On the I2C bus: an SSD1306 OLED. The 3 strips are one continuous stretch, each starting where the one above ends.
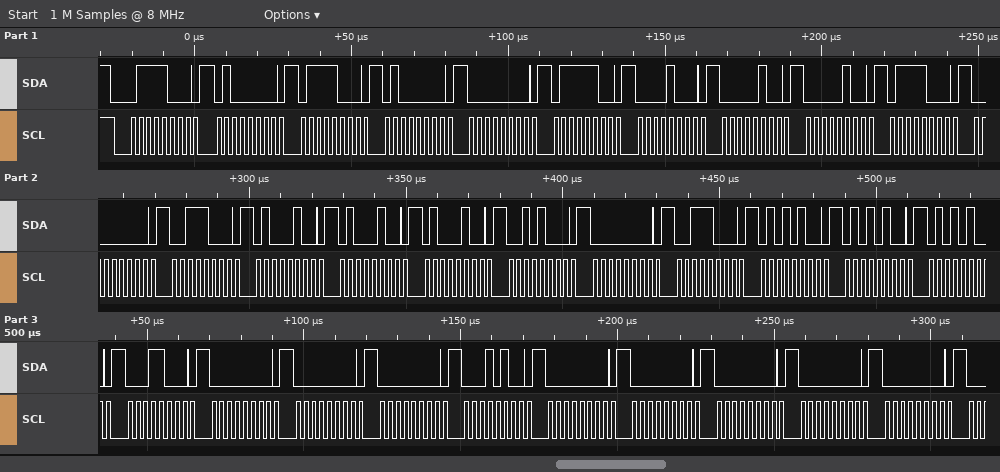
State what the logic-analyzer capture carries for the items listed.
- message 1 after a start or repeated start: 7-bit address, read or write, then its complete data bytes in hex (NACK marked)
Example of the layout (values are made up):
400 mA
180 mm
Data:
0x3C write: 40 78 40 00 7C 08 04 04 78 00 38 44 44 44 28 00 38 54 54 54 18 00 00 00 14 00 00 00 00 00
